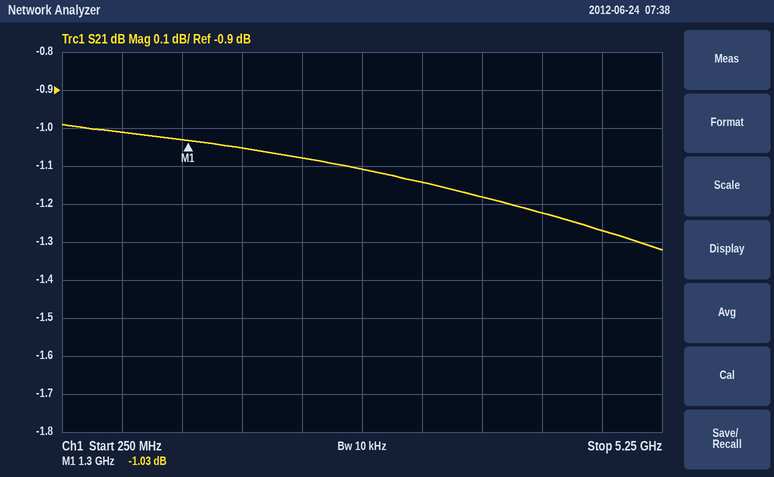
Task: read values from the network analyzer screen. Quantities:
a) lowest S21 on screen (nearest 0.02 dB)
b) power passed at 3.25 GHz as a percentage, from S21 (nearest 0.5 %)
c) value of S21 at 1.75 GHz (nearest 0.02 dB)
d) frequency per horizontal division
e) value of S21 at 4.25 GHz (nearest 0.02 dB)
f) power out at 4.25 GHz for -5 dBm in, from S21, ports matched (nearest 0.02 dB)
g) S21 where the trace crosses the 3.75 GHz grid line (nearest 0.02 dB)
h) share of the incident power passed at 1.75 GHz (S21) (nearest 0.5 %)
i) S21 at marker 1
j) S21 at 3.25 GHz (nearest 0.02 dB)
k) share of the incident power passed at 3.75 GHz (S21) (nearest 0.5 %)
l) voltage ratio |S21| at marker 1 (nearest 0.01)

-1.32 dB
77.0 %
-1.06 dB
500 MHz
-1.22 dB
-6.22 dBm
-1.18 dB
78.5 %
-1.03 dB
-1.14 dB
76.0 %
0.89
